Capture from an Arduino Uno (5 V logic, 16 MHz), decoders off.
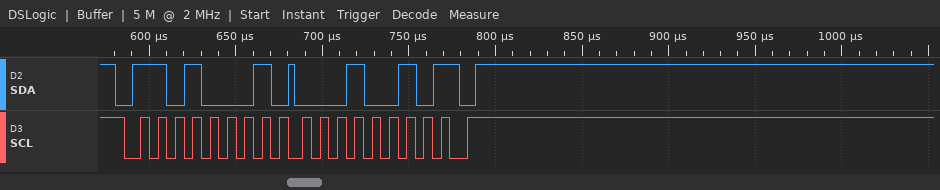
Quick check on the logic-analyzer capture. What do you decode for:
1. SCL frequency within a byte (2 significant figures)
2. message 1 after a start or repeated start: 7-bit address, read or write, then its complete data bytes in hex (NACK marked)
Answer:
100 kHz
0x68 read: 12 NACK
